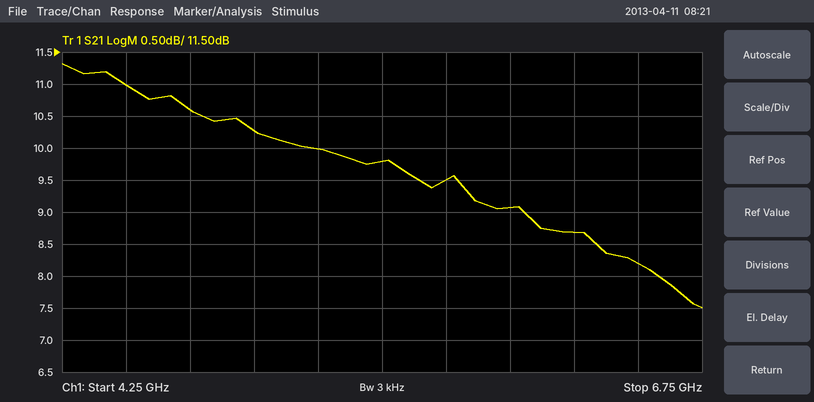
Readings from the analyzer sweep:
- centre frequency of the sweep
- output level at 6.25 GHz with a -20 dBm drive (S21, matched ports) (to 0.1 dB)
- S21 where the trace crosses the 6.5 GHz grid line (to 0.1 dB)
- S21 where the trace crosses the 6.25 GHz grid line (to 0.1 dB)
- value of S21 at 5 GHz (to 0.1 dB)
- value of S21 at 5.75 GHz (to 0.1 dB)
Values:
5.5 GHz
-11.3 dBm
8.2 dB
8.7 dB
10.3 dB
9.5 dB
